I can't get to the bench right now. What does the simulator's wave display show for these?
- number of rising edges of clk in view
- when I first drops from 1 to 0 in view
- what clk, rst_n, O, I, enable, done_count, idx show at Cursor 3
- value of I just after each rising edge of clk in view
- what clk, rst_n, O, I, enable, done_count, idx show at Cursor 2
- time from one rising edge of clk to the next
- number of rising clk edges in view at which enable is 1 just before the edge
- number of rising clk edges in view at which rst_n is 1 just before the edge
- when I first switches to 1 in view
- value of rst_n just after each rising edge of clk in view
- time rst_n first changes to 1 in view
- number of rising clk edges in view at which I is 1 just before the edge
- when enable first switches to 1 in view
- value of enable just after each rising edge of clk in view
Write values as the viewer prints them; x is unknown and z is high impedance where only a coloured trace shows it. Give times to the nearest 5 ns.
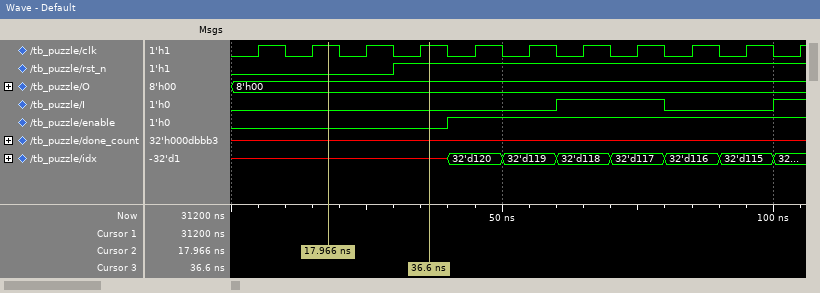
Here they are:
11
80 ns
clk=1, rst_n=1, O=8'h00, I=0, enable=0, done_count=x, idx=x
0 0 0 0 0 0 1 1 0 0 1
clk=1, rst_n=0, O=8'h00, I=0, enable=0, done_count=x, idx=x
10 ns
7
8
60 ns
0 0 0 1 1 1 1 1 1 1 1
30 ns
3
40 ns
0 0 0 0 1 1 1 1 1 1 1
